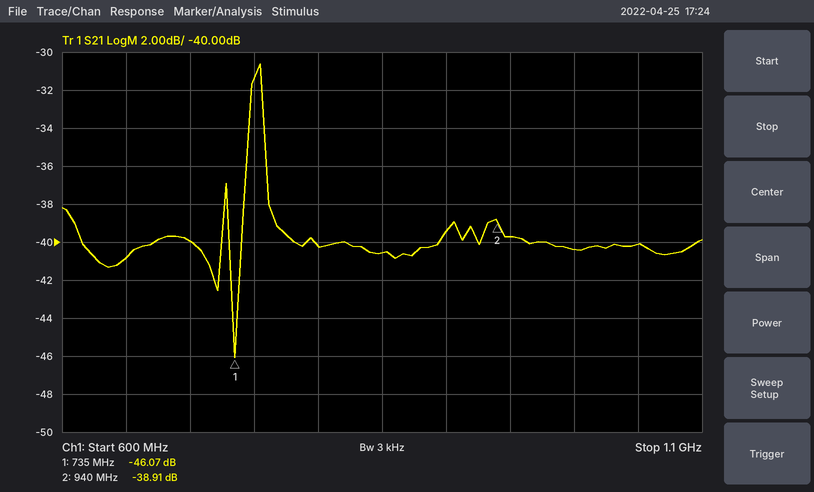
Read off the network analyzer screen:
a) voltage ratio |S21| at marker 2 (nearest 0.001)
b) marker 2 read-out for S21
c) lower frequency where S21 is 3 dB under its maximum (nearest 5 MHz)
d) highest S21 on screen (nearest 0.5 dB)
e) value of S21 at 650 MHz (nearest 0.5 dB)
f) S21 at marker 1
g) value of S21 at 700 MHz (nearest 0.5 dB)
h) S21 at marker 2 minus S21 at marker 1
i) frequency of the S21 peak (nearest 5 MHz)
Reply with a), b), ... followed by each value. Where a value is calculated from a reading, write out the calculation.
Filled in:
a) 10^(-38.91/20) ≈ 0.011
b) -38.91 dB
c) 745 MHz
d) -30.5 dB
e) -41.0 dB
f) -46.07 dB
g) -40.0 dB
h) -38.91 − (-46.07) = 7.16 dB
i) 755 MHz
